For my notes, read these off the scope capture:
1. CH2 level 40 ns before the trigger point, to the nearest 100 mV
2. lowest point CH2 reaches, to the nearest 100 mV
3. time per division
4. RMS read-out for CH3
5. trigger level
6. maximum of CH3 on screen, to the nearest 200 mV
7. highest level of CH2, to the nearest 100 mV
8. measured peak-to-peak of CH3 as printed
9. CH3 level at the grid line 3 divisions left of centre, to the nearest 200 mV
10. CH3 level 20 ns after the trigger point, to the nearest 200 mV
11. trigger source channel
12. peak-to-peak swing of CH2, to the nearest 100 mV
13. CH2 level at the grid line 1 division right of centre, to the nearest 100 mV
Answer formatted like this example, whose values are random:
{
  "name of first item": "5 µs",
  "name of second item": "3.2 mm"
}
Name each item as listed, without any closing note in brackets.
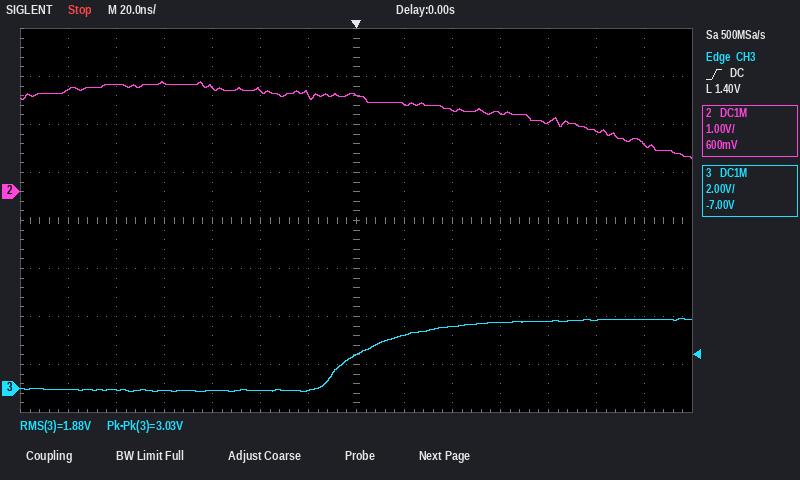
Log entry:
{
  "CH2 level 40 ns before the trigger point, to the nearest 100 mV": "2.1 V",
  "lowest point CH2 reaches, to the nearest 100 mV": "700 mV",
  "time per division": "20 ns",
  "RMS read-out for CH3": "1.88 V",
  "trigger level": "1.40 V",
  "maximum of CH3 on screen, to the nearest 200 mV": "3.0 V",
  "highest level of CH2, to the nearest 100 mV": "2.3 V",
  "measured peak-to-peak of CH3 as printed": "3.03 V",
  "CH3 level at the grid line 3 divisions left of centre, to the nearest 200 mV": "0.0 V",
  "CH3 level 20 ns after the trigger point, to the nearest 200 mV": "2.2 V",
  "trigger source channel": "CH3",
  "peak-to-peak swing of CH2, to the nearest 100 mV": "1.6 V",
  "CH2 level at the grid line 1 division right of centre, to the nearest 100 mV": "1.8 V"
}
